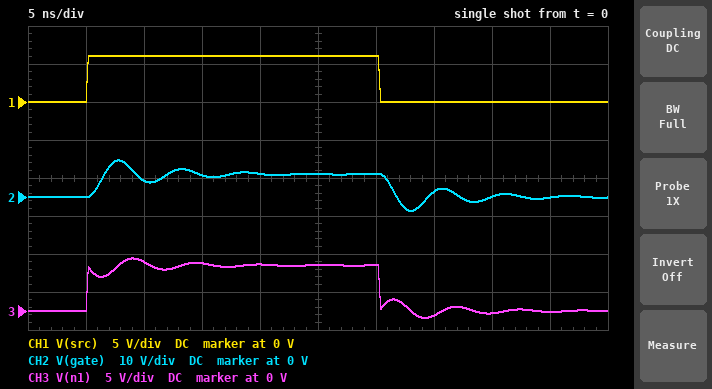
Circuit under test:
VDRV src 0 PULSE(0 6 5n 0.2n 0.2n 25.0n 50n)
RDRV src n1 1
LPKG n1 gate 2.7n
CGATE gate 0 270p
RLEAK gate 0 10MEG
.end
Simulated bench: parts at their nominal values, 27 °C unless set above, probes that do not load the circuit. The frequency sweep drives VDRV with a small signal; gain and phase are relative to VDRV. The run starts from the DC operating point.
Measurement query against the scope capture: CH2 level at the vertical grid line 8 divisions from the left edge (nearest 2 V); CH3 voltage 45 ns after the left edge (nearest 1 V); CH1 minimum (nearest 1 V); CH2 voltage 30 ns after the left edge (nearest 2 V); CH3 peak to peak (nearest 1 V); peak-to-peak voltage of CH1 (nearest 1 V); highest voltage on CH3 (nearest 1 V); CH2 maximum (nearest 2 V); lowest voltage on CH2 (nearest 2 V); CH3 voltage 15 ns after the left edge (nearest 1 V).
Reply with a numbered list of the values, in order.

1. 0 V
2. 0 V
3. 0 V
4. 6 V
5. 8 V
6. 6 V
7. 7 V
8. 10 V
9. -4 V
10. 6 V
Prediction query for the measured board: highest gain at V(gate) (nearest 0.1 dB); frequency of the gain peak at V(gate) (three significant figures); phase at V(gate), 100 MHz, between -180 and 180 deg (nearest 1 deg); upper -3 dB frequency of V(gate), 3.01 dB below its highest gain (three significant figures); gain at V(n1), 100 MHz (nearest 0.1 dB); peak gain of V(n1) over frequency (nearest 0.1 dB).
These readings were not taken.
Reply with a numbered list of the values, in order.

1. 10.1 dB
2. 182 MHz
3. -13 deg
4. 209 MHz
5. -0.2 dB
6. 0 dB
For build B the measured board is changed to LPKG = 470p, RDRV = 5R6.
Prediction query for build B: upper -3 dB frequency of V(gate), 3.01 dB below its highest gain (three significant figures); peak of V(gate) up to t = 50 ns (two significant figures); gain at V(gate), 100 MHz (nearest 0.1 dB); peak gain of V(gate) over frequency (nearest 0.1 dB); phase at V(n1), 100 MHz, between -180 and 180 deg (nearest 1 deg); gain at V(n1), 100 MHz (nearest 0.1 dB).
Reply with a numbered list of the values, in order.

1. 111 MHz
2. 6.0 V
3. -2.6 dB
4. 0 dB
5. -45 deg
6. -3.0 dB
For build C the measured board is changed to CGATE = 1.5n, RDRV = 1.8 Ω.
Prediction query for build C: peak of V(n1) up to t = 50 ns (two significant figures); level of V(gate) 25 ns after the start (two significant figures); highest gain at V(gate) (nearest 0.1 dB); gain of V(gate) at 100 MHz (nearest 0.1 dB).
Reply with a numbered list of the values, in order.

1. 6.2 V
2. 6.0 V
3. 0 dB
4. -5.1 dB
